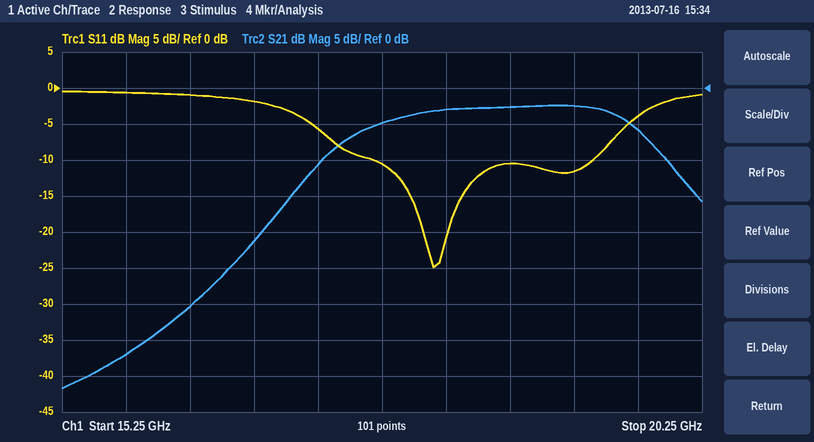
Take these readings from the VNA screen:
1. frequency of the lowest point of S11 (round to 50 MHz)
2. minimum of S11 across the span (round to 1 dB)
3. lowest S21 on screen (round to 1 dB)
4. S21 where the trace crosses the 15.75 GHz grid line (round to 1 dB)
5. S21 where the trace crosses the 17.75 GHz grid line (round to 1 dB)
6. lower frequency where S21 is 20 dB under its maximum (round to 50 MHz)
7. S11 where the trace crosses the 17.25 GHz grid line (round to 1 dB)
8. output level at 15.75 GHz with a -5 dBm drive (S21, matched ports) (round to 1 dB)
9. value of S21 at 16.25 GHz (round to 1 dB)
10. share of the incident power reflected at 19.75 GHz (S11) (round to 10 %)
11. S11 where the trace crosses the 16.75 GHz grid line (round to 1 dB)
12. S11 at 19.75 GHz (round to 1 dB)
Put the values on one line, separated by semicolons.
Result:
18.15 GHz; -25 dB; -42 dB; -37 dB; -5 dB; 16.70 GHz; -6 dB; -42 dBm; -30 dB; 40 %; -2 dB; -4 dB
